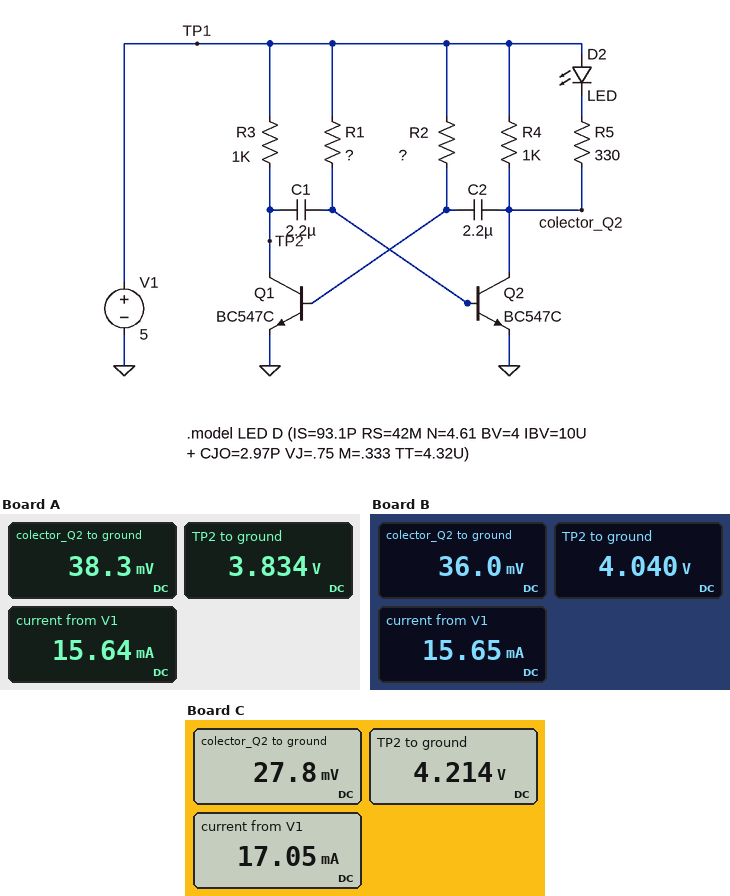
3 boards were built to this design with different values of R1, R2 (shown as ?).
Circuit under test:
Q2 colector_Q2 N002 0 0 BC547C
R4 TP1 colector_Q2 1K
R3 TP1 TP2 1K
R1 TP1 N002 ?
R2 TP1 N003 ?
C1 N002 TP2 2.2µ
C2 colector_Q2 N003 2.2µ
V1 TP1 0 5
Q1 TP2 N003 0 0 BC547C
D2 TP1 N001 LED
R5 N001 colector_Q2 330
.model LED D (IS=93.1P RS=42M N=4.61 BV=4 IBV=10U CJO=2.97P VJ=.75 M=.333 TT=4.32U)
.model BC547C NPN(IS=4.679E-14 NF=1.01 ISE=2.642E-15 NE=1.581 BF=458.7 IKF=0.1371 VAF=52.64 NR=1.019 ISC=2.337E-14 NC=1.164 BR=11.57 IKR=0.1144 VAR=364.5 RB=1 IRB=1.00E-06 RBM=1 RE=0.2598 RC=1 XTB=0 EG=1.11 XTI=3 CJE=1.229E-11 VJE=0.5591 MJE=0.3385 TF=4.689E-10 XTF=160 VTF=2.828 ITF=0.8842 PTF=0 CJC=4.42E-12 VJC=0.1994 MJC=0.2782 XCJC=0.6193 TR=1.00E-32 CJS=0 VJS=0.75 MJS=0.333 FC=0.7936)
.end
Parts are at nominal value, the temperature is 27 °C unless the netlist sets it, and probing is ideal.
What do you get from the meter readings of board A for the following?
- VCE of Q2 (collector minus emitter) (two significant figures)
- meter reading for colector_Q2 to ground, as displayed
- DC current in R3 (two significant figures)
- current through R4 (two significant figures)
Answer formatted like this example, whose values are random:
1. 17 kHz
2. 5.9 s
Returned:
1. 38 mV
2. 38.3 mV
3. 1.2 mA
4. 5.0 mA
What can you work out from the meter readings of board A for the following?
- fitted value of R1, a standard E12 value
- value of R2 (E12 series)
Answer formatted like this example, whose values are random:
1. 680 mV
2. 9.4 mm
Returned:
1. 3.9 kΩ
2. 1.8 MΩ
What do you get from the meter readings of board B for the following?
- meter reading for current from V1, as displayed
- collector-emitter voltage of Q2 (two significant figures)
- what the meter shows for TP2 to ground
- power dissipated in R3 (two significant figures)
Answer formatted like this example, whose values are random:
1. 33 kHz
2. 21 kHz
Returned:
1. 15.65 mA
2. 36 mV
3. 4.040 V
4. 920 µW
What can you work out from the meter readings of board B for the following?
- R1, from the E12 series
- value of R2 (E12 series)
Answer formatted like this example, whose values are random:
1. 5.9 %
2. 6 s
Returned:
1. 3.3 kΩ
2. 2.2 MΩ
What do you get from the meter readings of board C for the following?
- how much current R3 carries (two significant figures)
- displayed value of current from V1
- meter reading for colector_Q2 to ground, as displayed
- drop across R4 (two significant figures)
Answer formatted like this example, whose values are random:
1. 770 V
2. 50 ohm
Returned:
1. 790 µA
2. 17.05 mA
3. 27.8 mV
4. 5.0 V
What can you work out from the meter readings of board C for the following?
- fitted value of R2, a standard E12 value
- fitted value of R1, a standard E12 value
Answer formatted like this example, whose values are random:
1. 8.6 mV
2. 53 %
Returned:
1. 2.7 MΩ
2. 1.5 kΩ
